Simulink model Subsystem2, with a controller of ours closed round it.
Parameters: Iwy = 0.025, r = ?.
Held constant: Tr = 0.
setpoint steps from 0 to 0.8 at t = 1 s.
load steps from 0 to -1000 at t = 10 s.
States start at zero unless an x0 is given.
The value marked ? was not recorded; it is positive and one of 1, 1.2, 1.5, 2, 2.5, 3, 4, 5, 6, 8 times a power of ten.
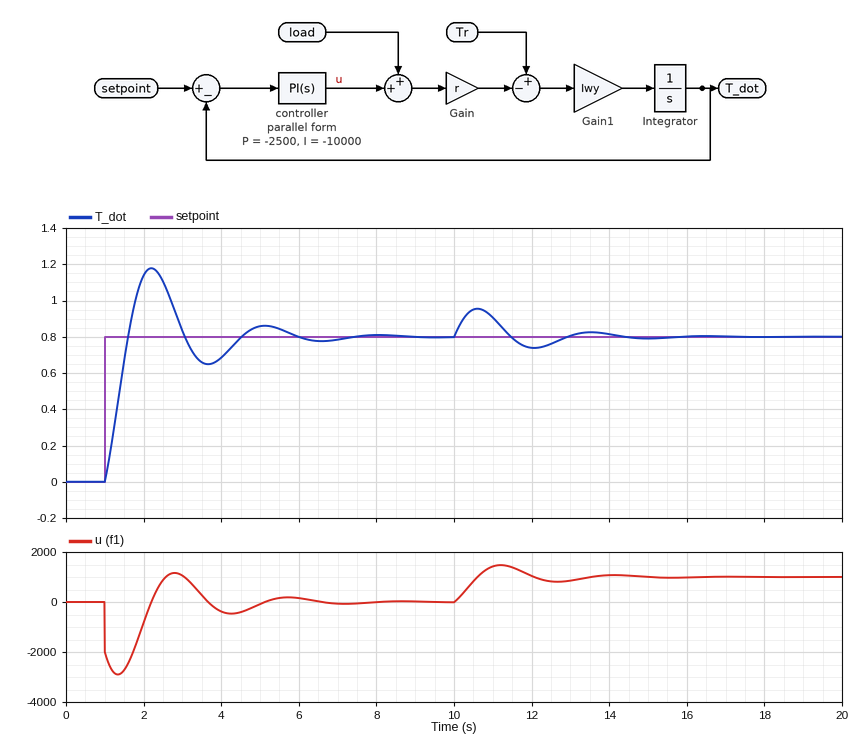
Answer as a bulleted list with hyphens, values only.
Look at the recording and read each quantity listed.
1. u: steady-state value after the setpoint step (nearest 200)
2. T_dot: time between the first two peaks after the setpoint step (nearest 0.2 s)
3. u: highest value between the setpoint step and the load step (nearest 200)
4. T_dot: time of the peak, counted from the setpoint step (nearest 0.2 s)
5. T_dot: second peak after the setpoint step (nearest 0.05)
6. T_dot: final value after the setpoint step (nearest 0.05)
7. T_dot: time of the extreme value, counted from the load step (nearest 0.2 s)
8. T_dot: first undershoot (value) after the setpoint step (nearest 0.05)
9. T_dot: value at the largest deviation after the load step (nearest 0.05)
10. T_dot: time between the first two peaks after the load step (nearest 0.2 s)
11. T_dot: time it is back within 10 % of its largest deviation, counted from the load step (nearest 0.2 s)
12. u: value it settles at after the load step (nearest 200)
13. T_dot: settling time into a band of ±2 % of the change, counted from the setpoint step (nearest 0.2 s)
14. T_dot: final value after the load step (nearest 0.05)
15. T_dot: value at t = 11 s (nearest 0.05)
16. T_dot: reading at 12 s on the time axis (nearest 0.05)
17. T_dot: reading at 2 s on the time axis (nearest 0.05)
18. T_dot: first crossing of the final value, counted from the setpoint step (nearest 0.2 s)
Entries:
- 0
- 3.0 s
- 1200
- 1.2 s
- 0.85
- 0.80
- 0.6 s
- 0.65
- 0.95
- 3.0 s
- 4.0 s
- 1000
- 6.0 s
- 0.80
- 0.90
- 0.75
- 1.15
- 0.6 s
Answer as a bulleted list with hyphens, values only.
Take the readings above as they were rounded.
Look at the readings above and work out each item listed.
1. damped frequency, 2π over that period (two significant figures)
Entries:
- 2.1 rad/s
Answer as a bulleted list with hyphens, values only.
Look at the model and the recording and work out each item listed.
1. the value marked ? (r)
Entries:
- 0.02
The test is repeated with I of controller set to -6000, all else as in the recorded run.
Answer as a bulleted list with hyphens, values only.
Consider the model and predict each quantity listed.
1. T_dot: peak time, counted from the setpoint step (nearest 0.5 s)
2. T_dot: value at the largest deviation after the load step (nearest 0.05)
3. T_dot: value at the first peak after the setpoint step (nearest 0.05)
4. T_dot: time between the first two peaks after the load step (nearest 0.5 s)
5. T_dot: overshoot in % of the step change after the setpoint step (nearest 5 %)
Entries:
- 1.5 s
- 1.00
- 1.10
- 4.0 s
- 40 %
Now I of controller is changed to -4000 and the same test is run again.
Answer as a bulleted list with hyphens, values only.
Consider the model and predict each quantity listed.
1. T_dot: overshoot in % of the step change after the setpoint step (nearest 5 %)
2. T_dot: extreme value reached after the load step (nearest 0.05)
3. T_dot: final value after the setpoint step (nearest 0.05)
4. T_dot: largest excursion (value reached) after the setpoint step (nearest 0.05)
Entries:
- 35 %
- 1.00
- 0.80
- 1.05
